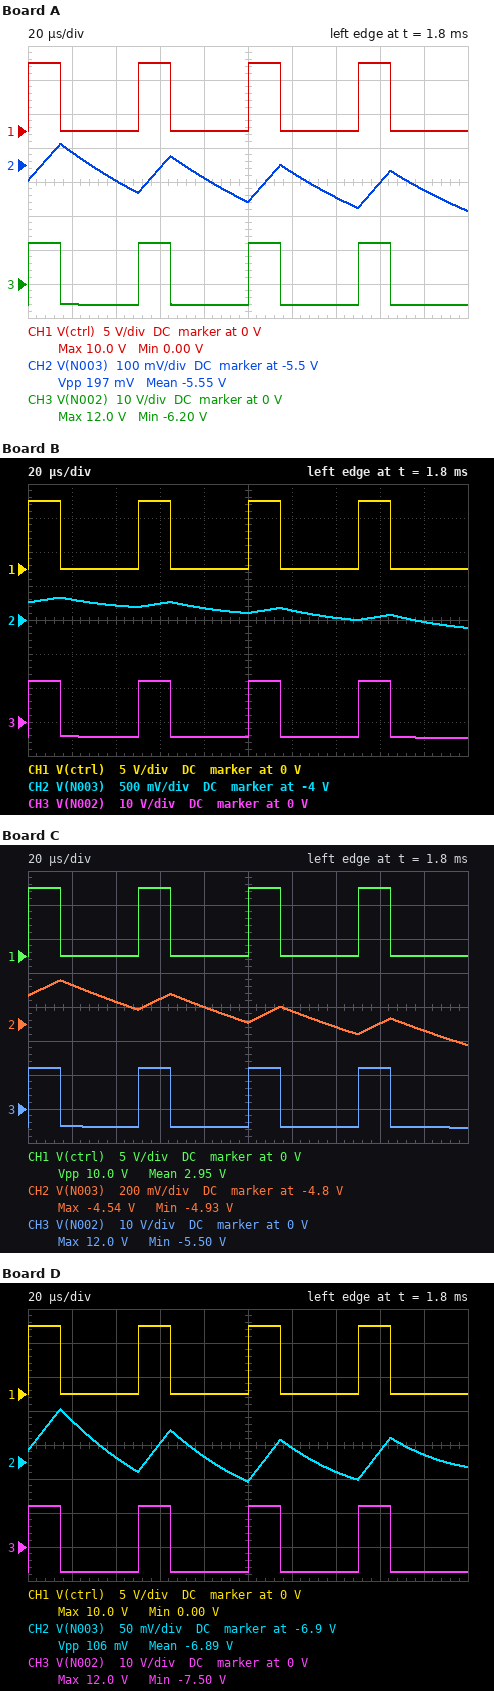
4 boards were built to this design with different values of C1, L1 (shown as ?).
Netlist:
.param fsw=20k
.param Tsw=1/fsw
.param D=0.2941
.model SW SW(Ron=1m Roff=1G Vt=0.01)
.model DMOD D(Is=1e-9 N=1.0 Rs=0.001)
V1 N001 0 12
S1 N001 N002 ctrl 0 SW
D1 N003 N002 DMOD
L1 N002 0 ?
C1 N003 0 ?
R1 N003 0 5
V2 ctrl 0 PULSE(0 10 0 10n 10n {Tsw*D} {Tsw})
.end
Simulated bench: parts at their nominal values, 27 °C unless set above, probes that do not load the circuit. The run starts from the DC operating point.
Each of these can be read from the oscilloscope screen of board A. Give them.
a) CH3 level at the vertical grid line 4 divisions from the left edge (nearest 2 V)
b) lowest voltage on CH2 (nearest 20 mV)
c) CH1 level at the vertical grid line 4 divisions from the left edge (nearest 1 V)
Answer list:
-6 V
-5.64 V
0 V
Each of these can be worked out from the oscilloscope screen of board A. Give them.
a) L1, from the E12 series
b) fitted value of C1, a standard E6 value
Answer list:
1.2 mH
150 µF
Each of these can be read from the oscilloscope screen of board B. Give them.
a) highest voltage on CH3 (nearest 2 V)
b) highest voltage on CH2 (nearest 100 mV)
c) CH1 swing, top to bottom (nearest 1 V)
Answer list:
12 V
-3.7 V
10 V
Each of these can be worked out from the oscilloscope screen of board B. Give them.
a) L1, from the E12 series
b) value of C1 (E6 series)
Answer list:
220 µH
150 µF
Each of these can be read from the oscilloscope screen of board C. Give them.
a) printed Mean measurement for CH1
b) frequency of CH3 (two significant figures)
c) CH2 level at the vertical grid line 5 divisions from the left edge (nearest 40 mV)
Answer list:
2.95 V
20 kHz
-4.80 V
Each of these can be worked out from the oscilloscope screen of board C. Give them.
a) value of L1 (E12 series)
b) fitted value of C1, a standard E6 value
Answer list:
1.8 mH
150 µF
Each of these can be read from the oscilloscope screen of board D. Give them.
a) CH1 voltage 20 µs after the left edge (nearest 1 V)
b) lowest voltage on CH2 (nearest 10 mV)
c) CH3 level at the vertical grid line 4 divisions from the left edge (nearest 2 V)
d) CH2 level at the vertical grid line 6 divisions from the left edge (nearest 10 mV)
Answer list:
0 V
-6.93 V
-8 V
-6.88 V
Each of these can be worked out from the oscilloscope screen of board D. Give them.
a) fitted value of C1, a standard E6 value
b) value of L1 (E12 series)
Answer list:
330 µF
560 µH
